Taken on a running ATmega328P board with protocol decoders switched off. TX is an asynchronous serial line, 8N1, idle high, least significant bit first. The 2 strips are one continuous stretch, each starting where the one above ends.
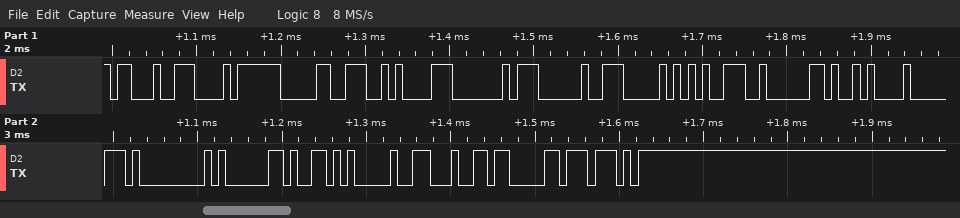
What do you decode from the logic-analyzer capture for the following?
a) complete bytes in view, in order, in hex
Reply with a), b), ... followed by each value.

a) 0x23 0xE8 0x30 0x0A 0x40 0x20 0x50 0x39 0x60 0x0A 0x70 0x00 0x81 0x59 0x90 0x64 0xB0 0xD7
